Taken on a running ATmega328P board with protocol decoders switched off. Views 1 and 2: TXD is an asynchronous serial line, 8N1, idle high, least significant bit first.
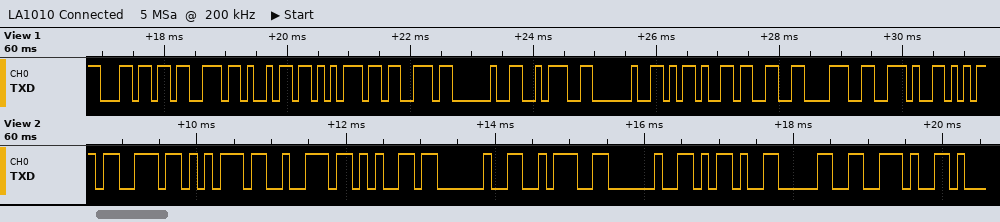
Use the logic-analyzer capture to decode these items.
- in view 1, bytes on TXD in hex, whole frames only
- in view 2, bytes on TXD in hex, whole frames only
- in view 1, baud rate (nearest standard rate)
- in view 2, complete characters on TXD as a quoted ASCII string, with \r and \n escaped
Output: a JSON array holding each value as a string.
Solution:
["6C 73 69 75 73 20 3A 20 2D 33 38 2E", "0x73 0x75 0x72 0x65 0x20 0x3A 0x20 0x2D 0x30 0x2E", "9600 baud", "\"sure : -0.\""]
